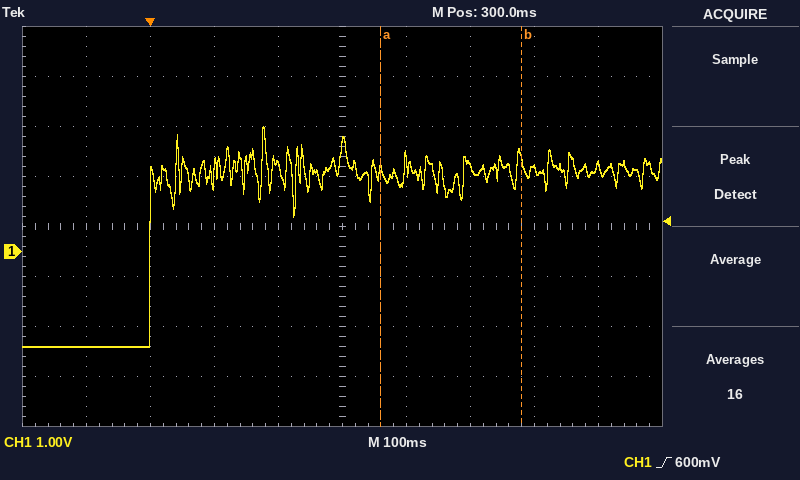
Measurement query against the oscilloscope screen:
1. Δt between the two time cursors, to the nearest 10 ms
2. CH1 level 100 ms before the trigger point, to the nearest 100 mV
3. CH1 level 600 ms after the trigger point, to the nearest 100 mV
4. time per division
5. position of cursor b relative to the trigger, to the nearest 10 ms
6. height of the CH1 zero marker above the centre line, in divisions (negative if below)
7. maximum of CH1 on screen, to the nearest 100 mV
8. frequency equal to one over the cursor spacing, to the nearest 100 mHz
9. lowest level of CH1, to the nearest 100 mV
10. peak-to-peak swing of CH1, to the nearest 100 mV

220 ms
-1.9 V
1.6 V
100 ms
+580 ms
-0.5 div
2.5 V
4.5 Hz
-1.9 V
4.4 V
